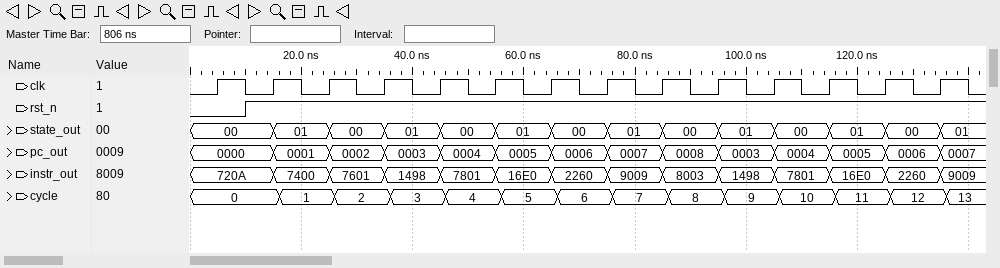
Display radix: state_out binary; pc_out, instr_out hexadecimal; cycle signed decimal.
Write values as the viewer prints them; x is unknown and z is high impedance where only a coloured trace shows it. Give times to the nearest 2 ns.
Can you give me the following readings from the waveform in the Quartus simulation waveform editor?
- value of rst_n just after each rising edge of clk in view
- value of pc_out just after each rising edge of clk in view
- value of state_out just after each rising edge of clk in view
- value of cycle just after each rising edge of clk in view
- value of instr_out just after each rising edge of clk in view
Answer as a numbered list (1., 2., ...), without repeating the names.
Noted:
1. 0 1 1 1 1 1 1 1 1 1 1 1 1 1
2. 0000, 0001, 0002, 0003, 0004, 0005, 0006, 0007, 0008, 0003, 0004, 0005, 0006, 0007
3. 00, 01, 00, 01, 00, 01, 00, 01, 00, 01, 00, 01, 00, 01
4. 0, 0, 1, 2, 3, 4, 5, 6, 7, 8, 9, 10, 11, 12
5. 720A, 7400, 7601, 1498, 7801, 16E0, 2260, 9009, 8003, 1498, 7801, 16E0, 2260, 9009
